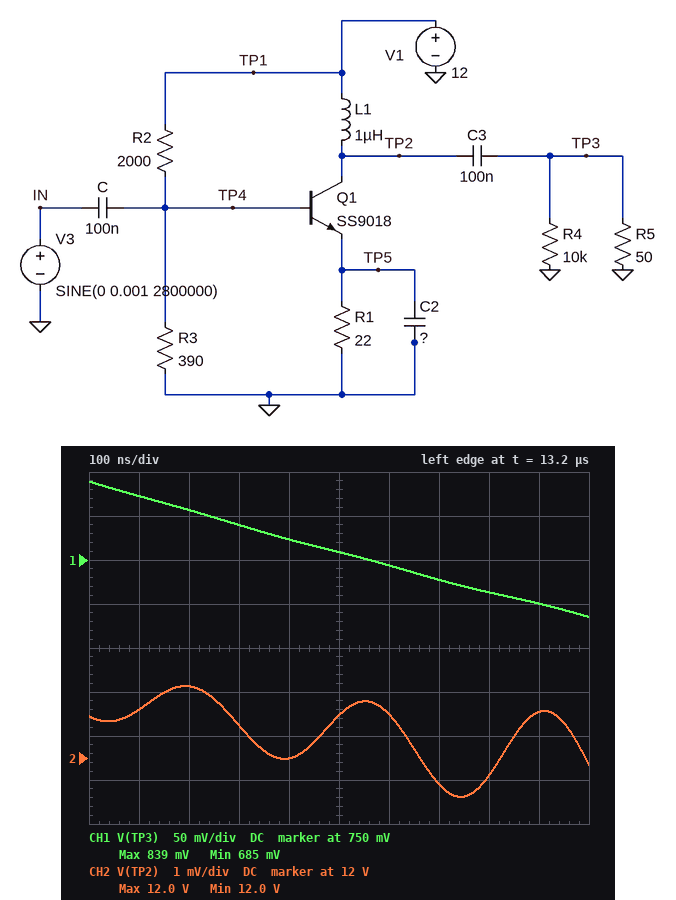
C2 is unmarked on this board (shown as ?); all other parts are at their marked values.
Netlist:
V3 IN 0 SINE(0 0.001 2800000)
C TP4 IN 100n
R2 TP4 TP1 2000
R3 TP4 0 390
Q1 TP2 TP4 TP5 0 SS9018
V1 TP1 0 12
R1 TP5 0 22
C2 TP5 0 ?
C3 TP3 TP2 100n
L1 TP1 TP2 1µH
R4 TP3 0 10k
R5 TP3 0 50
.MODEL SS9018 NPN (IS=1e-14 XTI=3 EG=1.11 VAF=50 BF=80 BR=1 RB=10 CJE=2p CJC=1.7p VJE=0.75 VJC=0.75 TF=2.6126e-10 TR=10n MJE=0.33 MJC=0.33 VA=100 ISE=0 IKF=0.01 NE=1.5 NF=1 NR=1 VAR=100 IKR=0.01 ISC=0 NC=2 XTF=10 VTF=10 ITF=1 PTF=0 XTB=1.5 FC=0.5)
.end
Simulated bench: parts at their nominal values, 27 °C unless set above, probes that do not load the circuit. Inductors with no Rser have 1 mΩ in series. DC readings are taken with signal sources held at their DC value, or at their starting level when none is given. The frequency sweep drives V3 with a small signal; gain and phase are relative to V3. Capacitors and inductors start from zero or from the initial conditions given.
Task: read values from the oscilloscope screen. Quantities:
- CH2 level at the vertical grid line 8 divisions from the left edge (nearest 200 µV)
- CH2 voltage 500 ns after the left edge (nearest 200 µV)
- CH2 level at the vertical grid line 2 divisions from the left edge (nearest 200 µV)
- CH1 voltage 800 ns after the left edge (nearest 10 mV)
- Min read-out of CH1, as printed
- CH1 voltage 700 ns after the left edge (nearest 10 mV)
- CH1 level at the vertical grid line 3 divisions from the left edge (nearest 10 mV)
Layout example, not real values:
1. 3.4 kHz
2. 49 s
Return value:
1. 12.0006 V
2. 12.0020 V
3. 12.0026 V
4. 710 mV
5. 685 mV
6. 730 mV
7. 790 mV
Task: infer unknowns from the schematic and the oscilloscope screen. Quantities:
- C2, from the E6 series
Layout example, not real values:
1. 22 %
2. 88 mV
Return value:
1. 150 nF
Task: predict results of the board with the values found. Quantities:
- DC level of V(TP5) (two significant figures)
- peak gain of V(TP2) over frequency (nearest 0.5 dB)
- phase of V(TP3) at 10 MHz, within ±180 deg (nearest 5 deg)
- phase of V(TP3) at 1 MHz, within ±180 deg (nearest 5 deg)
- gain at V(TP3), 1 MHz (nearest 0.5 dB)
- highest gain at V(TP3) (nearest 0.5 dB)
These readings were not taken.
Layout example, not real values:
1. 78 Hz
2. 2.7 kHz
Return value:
1. 720 mV
2. 26.5 dB
3. -145 deg
4. -65 deg
5. 7.5 dB
6. 26.5 dB
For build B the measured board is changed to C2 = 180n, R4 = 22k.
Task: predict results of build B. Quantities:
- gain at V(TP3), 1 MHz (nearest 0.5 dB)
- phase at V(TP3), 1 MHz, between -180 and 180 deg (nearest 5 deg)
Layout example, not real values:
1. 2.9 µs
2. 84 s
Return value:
1. 8.0 dB
2. -70 deg
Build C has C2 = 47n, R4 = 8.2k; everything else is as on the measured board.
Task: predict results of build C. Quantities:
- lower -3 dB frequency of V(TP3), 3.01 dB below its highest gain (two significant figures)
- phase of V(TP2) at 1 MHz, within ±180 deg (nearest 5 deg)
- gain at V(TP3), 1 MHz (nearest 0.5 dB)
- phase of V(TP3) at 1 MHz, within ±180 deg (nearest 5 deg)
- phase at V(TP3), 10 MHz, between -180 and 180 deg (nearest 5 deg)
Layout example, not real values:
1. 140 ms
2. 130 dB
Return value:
1. 7.2 MHz
2. -45 deg
3. 2.5 dB
4. -40 deg
5. -140 deg
